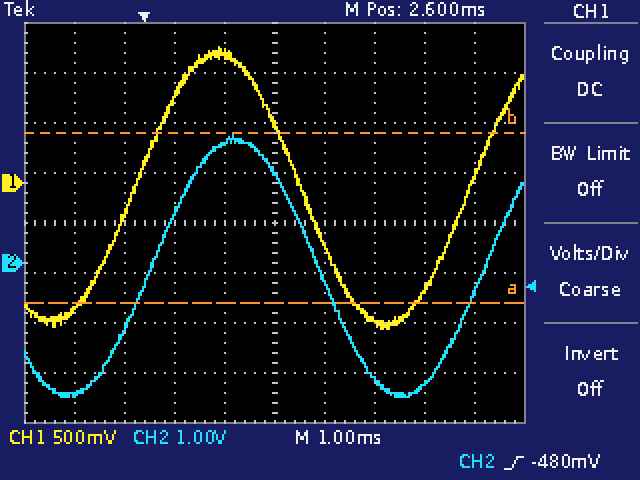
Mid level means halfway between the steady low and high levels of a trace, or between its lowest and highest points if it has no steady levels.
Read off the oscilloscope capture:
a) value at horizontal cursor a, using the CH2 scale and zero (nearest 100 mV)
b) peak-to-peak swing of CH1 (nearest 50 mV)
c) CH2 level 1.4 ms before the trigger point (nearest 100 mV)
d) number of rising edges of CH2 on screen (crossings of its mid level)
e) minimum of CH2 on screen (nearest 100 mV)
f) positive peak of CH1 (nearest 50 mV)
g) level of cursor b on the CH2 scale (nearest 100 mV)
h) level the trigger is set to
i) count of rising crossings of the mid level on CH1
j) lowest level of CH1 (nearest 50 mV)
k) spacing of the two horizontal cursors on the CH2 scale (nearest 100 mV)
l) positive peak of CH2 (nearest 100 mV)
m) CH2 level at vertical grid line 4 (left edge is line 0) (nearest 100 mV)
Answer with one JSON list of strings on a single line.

["-800 mV", "2.80 V", "-2.6 V", "2", "-2.7 V", "1.35 V", "2.6 V", "-480 mV", "2", "-1.45 V", "3.4 V", "2.6 V", "2.4 V"]
